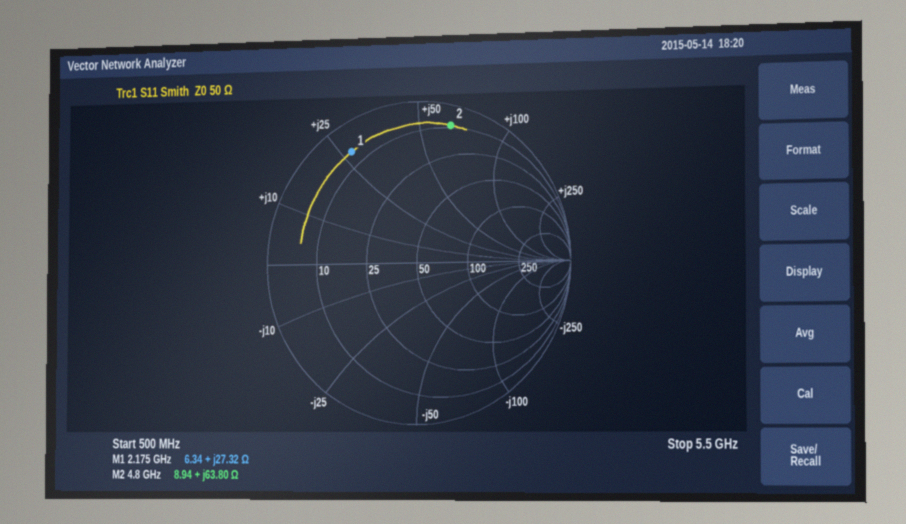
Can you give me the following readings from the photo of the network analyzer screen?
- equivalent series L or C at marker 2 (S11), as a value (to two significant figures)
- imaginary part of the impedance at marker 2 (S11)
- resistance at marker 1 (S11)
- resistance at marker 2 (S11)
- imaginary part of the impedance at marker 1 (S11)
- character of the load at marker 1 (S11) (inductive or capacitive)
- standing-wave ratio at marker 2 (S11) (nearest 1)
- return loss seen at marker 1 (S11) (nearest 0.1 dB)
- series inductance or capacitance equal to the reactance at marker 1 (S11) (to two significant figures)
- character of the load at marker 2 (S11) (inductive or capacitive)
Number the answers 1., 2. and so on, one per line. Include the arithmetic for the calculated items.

1. L = 63.8 Ω/(2π × 4.8 GHz) ≈ 2.1 nH
2. +63.80 Ω
3. 6.34 Ω
4. 8.94 Ω
5. +27.32 Ω
6. inductive
7. 15
8. 1.7 dB
9. L = 27.32 Ω/(2π × 2.175 GHz) ≈ 2.0 nH
10. inductive
